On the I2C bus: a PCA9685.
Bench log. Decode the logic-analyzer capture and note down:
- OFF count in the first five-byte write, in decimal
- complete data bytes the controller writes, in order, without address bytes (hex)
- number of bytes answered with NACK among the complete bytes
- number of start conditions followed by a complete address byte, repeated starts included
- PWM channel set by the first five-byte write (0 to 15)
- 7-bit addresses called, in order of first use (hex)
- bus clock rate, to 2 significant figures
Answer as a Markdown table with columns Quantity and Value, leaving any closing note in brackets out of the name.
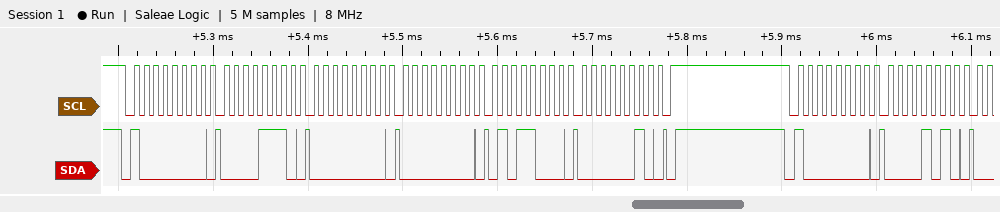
| Quantity | Value |
|---|---|
| OFF count in the first five-byte write, in decimal | 600 |
| complete data bytes the controller writes, in order, without address bytes | 0E 00 00 58 02 0A |
| number of bytes answered with NACK among the complete bytes | 0 |
| number of start conditions followed by a complete address byte, repeated starts included | 2 |
| PWM channel set by the first five-byte write | 2 |
| 7-bit addresses called, in order of first use | 0x40 |
| bus clock rate, to 2 significant figures | 100 kHz |
